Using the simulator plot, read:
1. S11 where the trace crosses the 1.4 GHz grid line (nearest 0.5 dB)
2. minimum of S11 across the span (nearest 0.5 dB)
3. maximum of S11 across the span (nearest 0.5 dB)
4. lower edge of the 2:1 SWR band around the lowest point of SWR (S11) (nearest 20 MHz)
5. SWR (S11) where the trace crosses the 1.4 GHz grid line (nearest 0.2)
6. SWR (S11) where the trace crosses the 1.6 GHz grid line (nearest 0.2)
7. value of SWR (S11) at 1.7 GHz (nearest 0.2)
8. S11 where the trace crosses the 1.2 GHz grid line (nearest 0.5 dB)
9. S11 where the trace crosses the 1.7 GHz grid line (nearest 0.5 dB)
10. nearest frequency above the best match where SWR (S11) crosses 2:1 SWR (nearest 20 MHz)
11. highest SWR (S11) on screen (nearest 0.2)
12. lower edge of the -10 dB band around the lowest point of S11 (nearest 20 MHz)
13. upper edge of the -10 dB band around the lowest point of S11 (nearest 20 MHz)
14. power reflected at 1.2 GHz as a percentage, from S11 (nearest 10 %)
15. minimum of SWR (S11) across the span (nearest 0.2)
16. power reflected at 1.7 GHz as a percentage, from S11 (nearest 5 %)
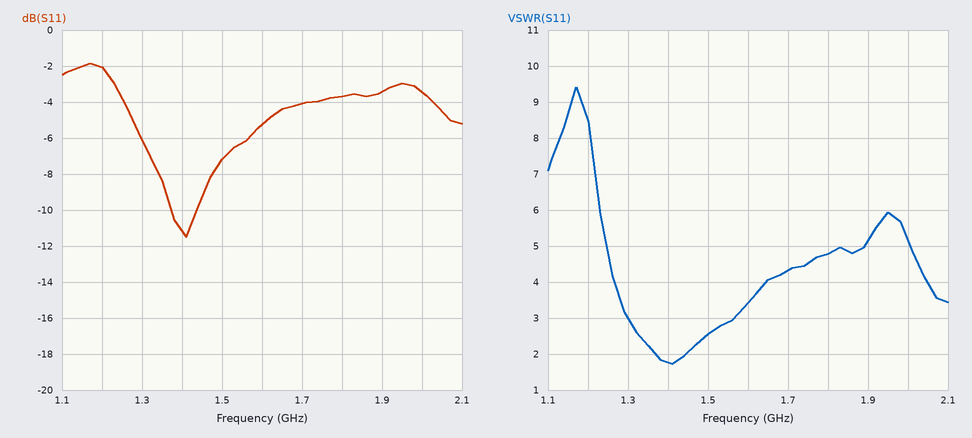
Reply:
-11.0 dB
-11.5 dB
-2.0 dB
1.36 GHz
1.8
3.4
4.4
-2.0 dB
-4.0 dB
1.44 GHz
9.4
1.38 GHz
1.44 GHz
60 %
1.8
40 %
